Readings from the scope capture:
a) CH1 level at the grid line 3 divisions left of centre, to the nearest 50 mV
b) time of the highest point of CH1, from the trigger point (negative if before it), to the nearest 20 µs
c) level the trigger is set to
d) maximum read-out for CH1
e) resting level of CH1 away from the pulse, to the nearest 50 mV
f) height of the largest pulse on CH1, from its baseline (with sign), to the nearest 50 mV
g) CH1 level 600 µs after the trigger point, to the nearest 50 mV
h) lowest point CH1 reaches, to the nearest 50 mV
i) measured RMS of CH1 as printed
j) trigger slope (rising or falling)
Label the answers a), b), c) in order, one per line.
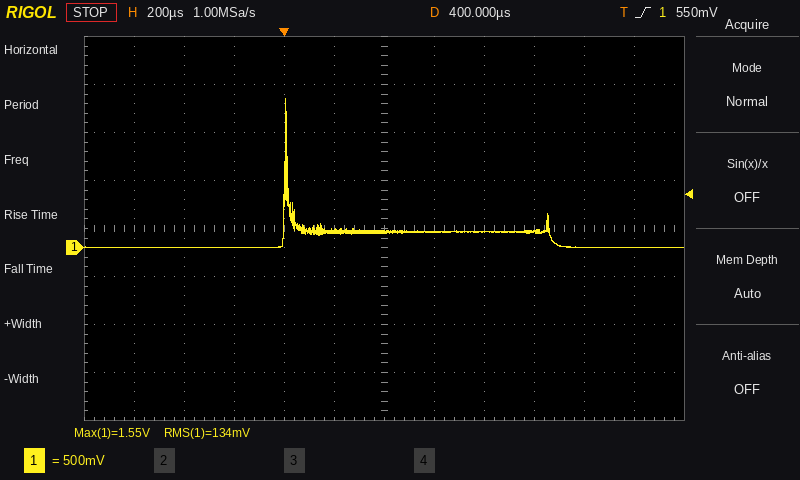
a) 0 mV
b) 0 µs
c) 550 mV
d) 1.55 V
e) 0 mV
f) +1.55 V
g) 150 mV
h) 0 mV
i) 134 mV
j) rising
